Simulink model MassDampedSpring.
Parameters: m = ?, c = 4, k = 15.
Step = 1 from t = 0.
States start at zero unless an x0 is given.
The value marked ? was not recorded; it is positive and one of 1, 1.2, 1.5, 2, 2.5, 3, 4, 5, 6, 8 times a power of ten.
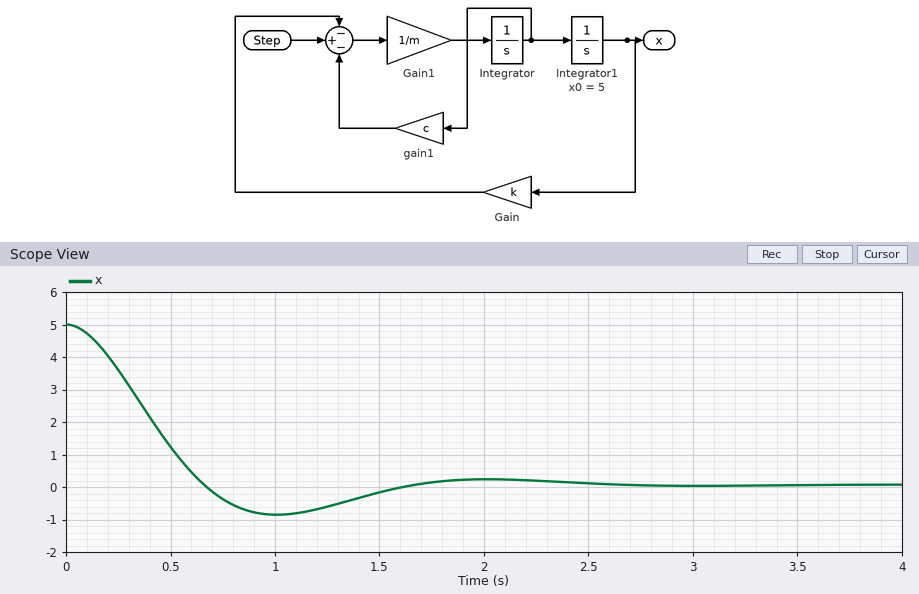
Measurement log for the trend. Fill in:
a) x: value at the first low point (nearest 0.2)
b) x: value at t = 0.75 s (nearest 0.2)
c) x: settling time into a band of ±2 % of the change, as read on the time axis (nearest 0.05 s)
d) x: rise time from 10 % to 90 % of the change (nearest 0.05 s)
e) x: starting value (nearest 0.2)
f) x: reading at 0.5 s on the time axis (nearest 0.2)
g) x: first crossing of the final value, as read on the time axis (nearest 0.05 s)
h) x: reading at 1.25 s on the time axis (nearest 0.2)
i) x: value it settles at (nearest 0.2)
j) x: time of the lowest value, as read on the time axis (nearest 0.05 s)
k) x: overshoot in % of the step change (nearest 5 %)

-0.8
-0.4
2.35 s
0.45 s
5.0
1.2
0.65 s
-0.6
0.0
1.00 s
20 %
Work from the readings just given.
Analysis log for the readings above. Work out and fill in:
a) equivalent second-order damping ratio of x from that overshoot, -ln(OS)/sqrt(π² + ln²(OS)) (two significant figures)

0.46
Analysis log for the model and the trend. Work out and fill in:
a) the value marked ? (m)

1.2
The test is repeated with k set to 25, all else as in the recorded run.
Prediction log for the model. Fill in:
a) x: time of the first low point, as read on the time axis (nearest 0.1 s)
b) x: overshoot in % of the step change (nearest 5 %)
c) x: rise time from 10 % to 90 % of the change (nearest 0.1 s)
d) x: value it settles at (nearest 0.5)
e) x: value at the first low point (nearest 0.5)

0.7 s
30 %
0.3 s
0.0
-1.5
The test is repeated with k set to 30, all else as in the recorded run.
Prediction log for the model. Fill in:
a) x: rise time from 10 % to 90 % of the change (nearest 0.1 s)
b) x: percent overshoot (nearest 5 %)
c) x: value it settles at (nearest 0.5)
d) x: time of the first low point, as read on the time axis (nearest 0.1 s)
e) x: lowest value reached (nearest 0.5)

0.3 s
35 %
0.0
0.7 s
-1.5
